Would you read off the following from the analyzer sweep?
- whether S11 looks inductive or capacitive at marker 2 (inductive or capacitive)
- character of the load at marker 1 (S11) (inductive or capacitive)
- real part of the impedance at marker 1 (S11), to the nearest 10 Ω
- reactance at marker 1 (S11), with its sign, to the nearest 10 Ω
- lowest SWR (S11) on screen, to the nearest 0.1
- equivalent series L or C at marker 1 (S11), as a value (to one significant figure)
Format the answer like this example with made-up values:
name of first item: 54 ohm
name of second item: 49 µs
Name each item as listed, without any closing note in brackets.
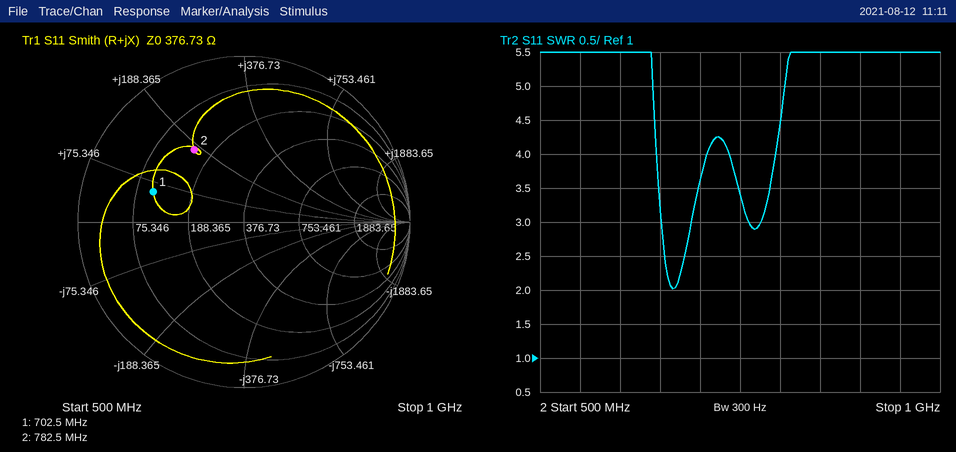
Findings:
whether S11 looks inductive or capacitive at marker 2: inductive
character of the load at marker 1 (S11): inductive
real part of the impedance at marker 1 (S11), to the nearest 10 Ω: 100 Ω
reactance at marker 1 (S11), with its sign, to the nearest 10 Ω: +60 Ω
lowest SWR (S11) on screen, to the nearest 0.1: 2.0
equivalent series L or C at marker 1 (S11), as a value: 10 nH
